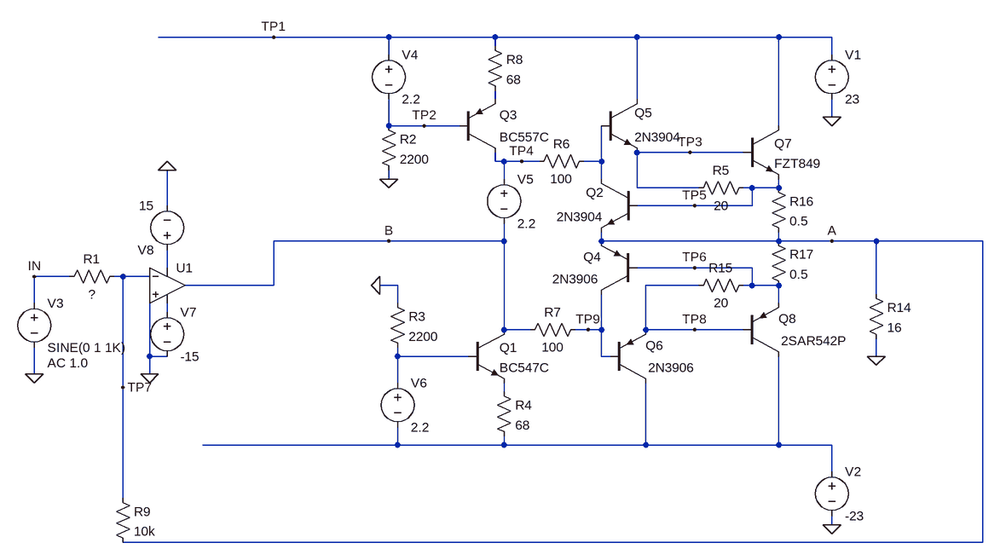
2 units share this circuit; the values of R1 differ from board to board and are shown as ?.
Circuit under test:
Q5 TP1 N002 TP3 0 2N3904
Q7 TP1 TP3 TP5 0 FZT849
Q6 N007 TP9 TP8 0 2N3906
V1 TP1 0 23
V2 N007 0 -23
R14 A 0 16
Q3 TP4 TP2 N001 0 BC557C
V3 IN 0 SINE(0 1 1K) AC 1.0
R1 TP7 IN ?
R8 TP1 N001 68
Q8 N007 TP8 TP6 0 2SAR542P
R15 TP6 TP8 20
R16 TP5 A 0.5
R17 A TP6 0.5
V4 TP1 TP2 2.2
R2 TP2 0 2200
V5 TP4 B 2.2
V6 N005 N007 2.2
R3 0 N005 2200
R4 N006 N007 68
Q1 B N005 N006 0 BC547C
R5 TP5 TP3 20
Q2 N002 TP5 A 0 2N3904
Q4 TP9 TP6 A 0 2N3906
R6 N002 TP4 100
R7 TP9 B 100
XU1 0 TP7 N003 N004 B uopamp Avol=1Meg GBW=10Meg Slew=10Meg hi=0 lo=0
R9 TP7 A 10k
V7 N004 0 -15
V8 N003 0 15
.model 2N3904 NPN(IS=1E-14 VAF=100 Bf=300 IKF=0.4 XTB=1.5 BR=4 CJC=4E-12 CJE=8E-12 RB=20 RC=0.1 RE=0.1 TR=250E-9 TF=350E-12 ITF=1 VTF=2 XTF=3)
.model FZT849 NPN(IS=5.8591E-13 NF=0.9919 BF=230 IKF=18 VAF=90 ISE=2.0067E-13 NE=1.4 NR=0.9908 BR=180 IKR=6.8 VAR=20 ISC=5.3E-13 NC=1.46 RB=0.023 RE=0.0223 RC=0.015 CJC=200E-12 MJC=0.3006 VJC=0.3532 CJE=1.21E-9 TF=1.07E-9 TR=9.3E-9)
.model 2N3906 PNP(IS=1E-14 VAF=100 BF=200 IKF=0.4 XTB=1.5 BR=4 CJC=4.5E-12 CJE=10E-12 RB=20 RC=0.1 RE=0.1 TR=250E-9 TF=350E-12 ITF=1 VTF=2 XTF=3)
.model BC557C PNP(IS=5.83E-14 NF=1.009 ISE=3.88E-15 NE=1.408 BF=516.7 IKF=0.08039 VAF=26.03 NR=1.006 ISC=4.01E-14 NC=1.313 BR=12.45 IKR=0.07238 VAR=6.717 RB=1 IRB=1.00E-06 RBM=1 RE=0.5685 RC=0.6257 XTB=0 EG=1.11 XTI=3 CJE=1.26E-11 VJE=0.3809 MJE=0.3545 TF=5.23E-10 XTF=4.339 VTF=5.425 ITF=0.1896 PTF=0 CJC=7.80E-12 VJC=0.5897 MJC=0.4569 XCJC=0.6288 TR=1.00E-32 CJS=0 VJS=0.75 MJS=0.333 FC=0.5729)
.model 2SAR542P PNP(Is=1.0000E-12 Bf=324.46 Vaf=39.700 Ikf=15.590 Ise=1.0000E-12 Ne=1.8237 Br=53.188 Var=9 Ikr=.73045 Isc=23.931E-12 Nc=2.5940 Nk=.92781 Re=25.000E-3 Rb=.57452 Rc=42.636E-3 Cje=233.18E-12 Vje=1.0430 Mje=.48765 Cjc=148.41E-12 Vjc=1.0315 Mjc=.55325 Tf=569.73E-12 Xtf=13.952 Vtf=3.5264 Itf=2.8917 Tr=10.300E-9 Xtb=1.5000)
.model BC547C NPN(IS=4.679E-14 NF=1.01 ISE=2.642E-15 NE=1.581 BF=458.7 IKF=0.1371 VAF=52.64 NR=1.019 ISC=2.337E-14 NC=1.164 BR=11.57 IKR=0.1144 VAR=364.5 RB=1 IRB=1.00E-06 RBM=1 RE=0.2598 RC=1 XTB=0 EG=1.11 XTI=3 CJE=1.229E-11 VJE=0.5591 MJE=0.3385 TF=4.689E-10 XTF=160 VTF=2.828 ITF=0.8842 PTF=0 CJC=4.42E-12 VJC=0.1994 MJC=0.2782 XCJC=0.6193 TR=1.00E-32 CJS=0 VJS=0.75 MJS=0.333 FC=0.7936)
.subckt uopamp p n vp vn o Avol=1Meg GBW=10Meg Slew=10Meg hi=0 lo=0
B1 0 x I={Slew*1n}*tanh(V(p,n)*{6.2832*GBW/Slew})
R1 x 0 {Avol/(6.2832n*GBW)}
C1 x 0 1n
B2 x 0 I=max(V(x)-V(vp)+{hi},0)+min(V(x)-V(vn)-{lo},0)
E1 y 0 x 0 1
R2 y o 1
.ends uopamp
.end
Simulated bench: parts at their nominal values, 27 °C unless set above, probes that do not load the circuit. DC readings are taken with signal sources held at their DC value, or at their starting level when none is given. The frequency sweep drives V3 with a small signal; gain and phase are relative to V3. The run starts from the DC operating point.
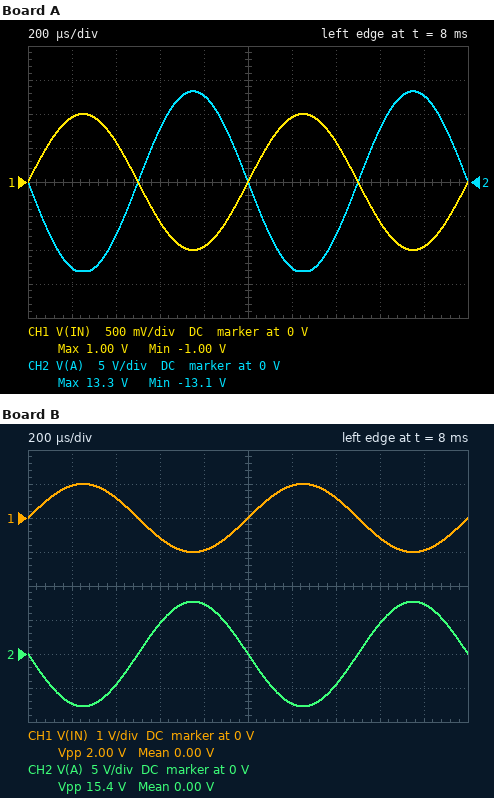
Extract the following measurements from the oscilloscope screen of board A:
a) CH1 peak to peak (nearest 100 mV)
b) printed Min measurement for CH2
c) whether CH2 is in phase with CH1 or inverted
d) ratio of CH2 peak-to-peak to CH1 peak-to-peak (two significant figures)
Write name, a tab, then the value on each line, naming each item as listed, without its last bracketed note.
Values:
CH1 peak to peak	2.0 V
printed Min measurement for CH2	-13.1 V
whether CH2 is in phase with CH1 or inverted	inverted
ratio of CH2 peak-to-peak to CH1 peak-to-peak	13
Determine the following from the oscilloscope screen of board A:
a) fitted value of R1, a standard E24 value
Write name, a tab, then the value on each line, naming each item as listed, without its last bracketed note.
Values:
fitted value of R1, a standard E24 value	750 Ω
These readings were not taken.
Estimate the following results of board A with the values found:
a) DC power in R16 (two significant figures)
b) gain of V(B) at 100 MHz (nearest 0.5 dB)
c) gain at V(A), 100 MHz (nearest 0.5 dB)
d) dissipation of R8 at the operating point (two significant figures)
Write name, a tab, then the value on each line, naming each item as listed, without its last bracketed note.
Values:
DC power in R16	160 µW
gain of V(B) at 100 MHz	-20.5 dB
gain at V(A), 100 MHz	-23.0 dB
dissipation of R8 at the operating point	33 mW
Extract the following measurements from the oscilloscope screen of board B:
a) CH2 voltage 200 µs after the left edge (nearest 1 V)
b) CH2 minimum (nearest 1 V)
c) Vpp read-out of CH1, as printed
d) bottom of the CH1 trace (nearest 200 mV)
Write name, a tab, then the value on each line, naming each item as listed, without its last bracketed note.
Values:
CH2 voltage 200 µs after the left edge	-7 V
CH2 minimum	-8 V
Vpp read-out of CH1, as printed	2.00 V
bottom of the CH1 trace	-1.0 V
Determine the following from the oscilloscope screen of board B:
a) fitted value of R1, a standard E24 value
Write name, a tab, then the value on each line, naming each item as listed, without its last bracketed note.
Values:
fitted value of R1, a standard E24 value	1.3 kΩ
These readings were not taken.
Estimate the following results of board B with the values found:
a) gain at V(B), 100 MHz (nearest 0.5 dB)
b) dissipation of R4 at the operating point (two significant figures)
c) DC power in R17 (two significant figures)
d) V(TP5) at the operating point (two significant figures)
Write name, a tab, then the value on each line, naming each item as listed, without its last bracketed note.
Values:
gain at V(B), 100 MHz	-21.0 dB
dissipation of R4 at the operating point	33 mW
DC power in R17	160 µW
V(TP5) at the operating point	8.9 mV
